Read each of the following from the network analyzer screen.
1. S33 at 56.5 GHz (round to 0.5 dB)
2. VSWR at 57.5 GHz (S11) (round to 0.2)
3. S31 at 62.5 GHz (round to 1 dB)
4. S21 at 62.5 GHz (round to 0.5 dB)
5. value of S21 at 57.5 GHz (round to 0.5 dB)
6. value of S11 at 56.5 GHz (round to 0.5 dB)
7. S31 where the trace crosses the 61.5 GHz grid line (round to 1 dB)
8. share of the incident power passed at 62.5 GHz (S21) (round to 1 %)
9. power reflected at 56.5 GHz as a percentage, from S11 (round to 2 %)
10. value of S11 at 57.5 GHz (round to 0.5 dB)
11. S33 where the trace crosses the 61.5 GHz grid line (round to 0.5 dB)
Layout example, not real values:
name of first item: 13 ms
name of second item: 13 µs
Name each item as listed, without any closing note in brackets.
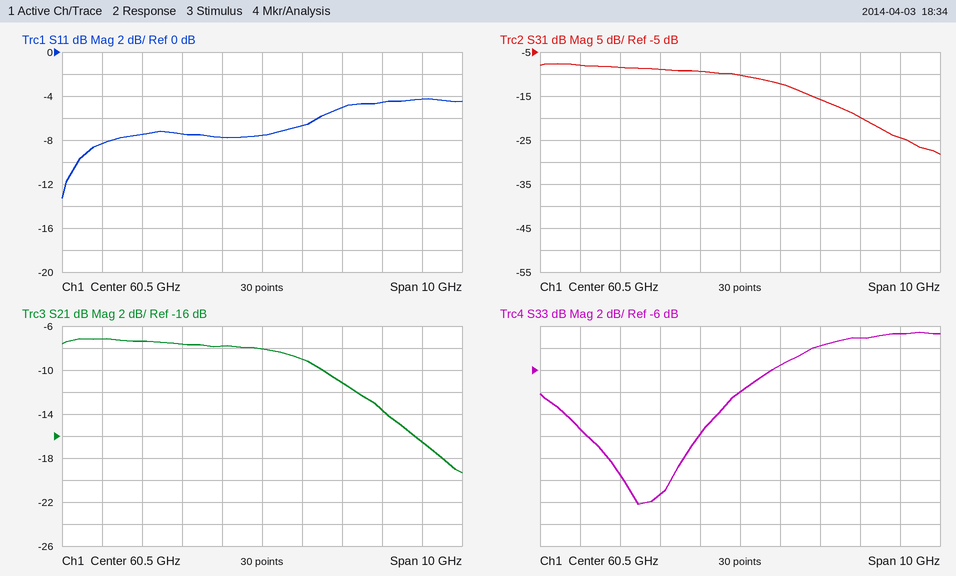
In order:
S33 at 56.5 GHz: -11.5 dB
VSWR at 57.5 GHz (S11): 2.4
S31 at 62.5 GHz: -16 dB
S21 at 62.5 GHz: -11.0 dB
value of S21 at 57.5 GHz: -7.5 dB
value of S11 at 56.5 GHz: -8.5 dB
S31 where the trace crosses the 61.5 GHz grid line: -12 dB
share of the incident power passed at 62.5 GHz (S21): 8 %
power reflected at 56.5 GHz as a percentage, from S11: 14 %
value of S11 at 57.5 GHz: -7.5 dB
S33 where the trace crosses the 61.5 GHz grid line: -5.5 dB
